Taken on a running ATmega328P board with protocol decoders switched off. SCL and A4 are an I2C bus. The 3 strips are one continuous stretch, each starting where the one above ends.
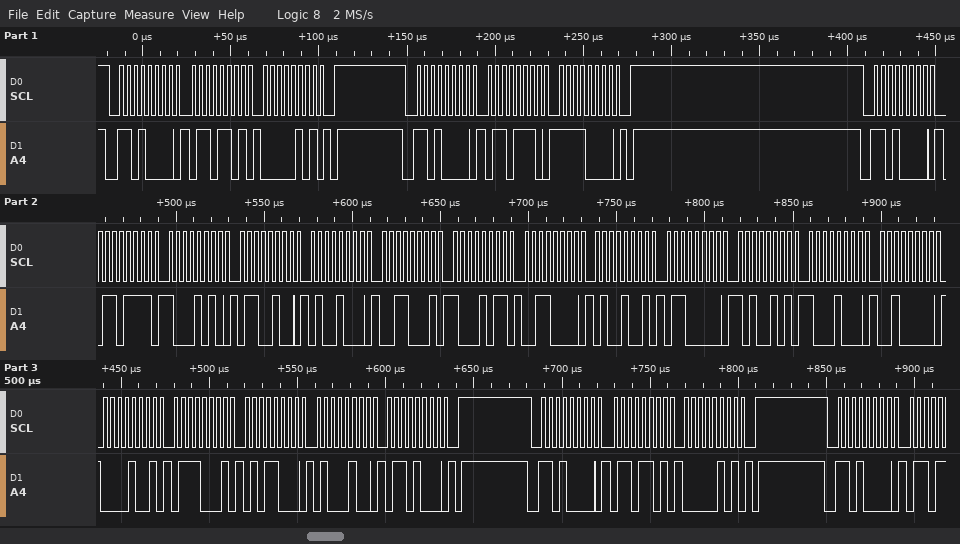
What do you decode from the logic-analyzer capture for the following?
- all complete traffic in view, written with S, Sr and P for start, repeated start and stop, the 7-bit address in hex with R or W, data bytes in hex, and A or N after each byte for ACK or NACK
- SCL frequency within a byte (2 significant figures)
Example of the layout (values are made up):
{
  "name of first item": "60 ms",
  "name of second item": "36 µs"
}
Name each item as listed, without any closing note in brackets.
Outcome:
{
  "all complete traffic in view, written with S, Sr and P for start, repeated start and stop, the 7-bit address in hex with R or W, data bytes in hex, and A or N after each byte for ACK or NACK": "S 68W A 6D A 05 A P S 68W A 6E A F0 A P S 68W A 6F A 8A A 64 A 48 A 31 A 8B A 30 A 49 A 60 A A5 A 88 A 20 A 09 A 71 A 58 A 44 A 68 A P S 68W A 6D A 05 A P S 68W A",
  "SCL frequency within a byte": "250 kHz"
}
